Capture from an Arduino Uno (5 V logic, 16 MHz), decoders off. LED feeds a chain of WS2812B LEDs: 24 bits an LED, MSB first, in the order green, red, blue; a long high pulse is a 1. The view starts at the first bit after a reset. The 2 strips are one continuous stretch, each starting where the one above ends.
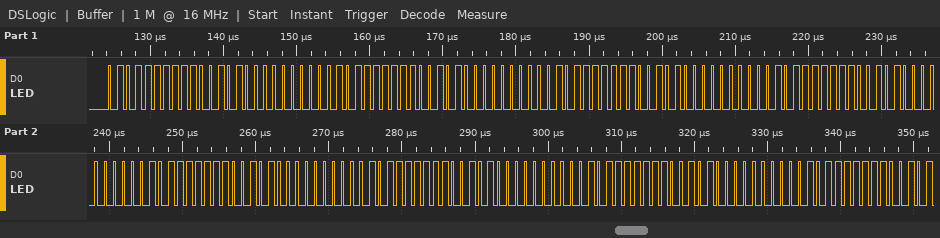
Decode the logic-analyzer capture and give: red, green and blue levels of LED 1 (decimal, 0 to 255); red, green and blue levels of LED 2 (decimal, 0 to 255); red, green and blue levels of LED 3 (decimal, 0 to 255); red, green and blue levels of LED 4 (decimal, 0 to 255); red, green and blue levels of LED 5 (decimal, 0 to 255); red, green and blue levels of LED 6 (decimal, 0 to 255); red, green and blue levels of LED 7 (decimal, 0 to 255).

202, 95, 0
202, 95, 0
202, 95, 0
202, 95, 0
202, 95, 0
202, 95, 0
202, 95, 0
